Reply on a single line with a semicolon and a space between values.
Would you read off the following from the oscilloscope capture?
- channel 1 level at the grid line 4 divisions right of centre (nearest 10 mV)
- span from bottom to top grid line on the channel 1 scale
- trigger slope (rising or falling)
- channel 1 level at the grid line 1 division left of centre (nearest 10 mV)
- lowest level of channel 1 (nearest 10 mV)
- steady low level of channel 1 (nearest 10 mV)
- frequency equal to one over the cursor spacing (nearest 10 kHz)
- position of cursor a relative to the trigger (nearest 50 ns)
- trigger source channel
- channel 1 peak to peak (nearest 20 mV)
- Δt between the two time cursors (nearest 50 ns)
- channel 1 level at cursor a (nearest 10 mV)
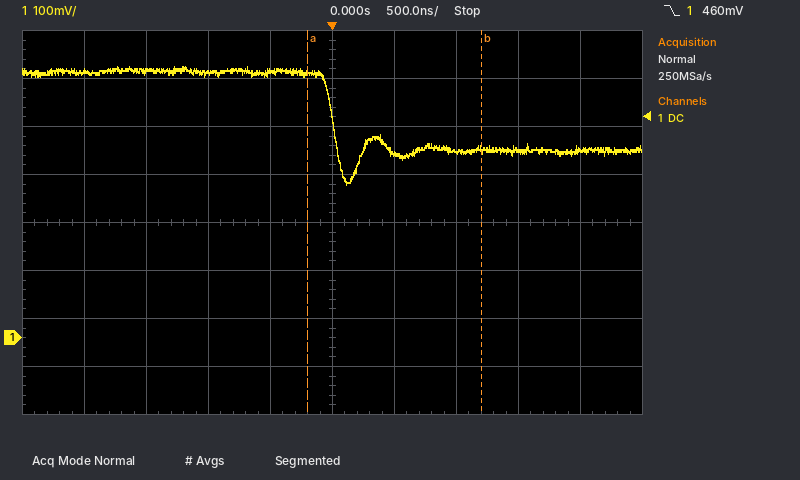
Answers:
390 mV; 800 mV; falling; 550 mV; 320 mV; 390 mV; 710 kHz; -200 ns; channel 1; 240 mV; 1.40 µs; 550 mV
